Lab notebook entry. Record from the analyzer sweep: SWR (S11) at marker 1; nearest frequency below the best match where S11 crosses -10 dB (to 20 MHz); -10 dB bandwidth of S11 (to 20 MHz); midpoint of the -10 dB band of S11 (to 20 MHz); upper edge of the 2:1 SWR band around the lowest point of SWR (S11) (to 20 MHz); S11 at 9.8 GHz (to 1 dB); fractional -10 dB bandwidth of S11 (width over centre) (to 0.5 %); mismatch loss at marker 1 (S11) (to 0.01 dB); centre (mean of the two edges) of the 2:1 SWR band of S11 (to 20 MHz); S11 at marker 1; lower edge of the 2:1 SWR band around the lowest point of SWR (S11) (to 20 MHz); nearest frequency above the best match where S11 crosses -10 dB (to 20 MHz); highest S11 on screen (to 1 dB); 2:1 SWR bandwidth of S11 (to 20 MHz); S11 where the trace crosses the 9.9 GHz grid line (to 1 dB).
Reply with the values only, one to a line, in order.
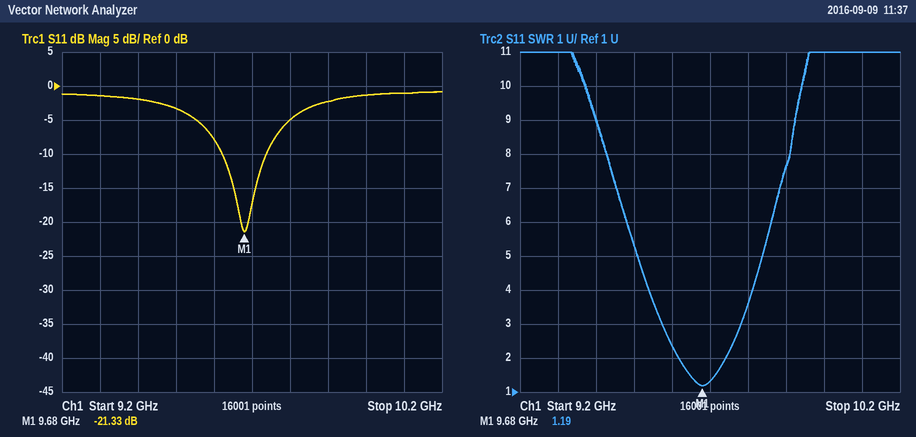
1.19
9.62 GHz
120 MHz
9.68 GHz
9.74 GHz
-5 dB
1.0 %
0.03 dB
9.68 GHz
-21.33 dB
9.62 GHz
9.74 GHz
-1 dB
120 MHz
-2 dB
